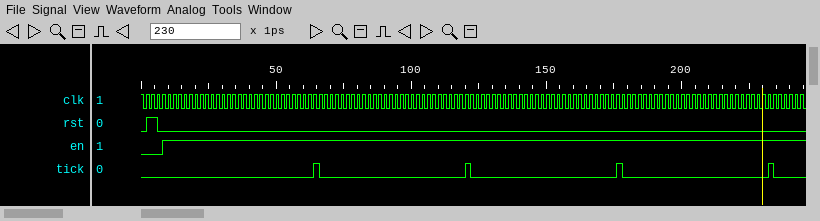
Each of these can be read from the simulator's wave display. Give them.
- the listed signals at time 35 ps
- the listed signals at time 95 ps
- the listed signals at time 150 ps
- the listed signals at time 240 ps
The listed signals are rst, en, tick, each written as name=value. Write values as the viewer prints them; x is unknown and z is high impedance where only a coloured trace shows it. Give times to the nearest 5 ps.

rst=0, en=1, tick=0
rst=0, en=1, tick=0
rst=0, en=1, tick=0
rst=0, en=1, tick=0
